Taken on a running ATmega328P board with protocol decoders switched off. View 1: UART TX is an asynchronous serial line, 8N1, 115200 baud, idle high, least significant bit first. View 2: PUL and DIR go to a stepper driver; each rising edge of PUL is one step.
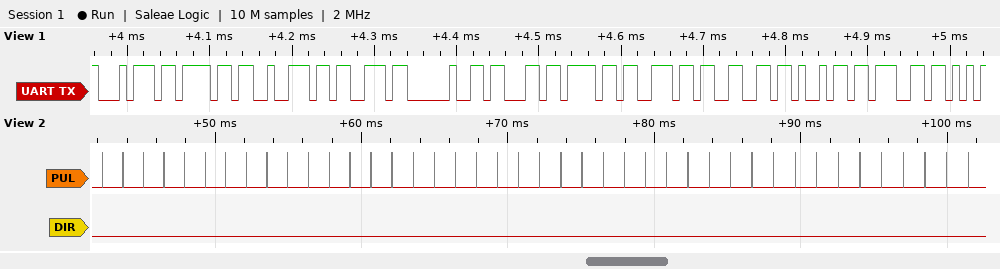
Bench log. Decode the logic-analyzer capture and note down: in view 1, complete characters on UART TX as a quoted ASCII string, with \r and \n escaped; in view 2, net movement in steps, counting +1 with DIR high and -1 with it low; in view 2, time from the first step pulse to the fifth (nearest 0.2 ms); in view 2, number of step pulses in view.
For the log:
"tors config"
-42
5.6 ms
42
